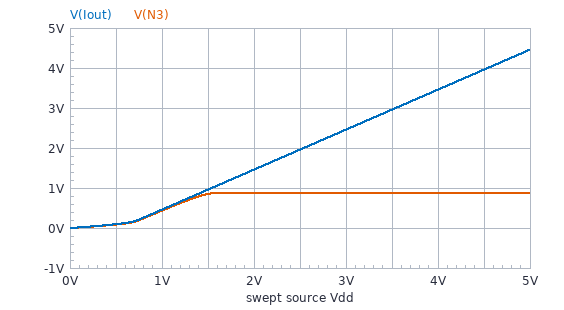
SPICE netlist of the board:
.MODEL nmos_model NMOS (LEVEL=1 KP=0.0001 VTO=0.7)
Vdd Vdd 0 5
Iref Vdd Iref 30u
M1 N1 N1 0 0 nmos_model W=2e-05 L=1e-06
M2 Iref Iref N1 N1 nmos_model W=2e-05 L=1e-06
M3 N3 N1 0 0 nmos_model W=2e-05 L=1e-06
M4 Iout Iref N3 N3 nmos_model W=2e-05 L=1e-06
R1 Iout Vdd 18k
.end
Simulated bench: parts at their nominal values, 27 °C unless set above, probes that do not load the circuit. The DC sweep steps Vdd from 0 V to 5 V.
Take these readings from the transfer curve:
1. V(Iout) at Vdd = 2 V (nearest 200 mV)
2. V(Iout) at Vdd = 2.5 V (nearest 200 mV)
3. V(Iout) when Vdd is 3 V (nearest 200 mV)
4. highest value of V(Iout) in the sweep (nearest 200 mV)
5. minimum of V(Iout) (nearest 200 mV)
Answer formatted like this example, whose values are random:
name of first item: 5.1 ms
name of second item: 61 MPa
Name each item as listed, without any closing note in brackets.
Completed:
V(Iout) at Vdd = 2 V: 1.4 V
V(Iout) at Vdd = 2.5 V: 2.0 V
V(Iout) when Vdd is 3 V: 2.4 V
highest value of V(Iout) in the sweep: 4.4 V
minimum of V(Iout): 0 V
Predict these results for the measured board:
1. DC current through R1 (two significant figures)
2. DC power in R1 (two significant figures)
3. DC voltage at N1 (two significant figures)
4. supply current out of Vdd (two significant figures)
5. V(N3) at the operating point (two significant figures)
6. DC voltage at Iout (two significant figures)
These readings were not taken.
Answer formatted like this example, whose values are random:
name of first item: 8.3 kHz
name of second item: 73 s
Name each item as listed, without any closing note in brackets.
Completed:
DC current through R1: 30 µA
DC power in R1: 16 µW
DC voltage at N1: 870 mV
supply current out of Vdd: 60 µA
V(N3) at the operating point: 870 mV
DC voltage at Iout: 4.5 V
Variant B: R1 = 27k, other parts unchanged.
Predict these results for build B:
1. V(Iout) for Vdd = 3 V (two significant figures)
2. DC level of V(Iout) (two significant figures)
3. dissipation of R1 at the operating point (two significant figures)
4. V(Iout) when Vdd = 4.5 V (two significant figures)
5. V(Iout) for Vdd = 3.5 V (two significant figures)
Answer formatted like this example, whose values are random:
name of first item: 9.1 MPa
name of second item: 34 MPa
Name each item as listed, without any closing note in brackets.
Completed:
V(Iout) for Vdd = 3 V: 2.2 V
DC level of V(Iout): 4.2 V
dissipation of R1 at the operating point: 24 µW
V(Iout) when Vdd = 4.5 V: 3.7 V
V(Iout) for Vdd = 3.5 V: 2.7 V
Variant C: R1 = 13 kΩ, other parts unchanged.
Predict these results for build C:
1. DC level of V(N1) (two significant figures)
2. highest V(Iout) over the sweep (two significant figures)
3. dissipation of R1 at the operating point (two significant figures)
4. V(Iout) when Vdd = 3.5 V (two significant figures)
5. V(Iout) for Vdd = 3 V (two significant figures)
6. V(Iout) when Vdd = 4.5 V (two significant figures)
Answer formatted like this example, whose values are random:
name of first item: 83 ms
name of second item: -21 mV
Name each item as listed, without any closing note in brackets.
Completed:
DC level of V(N1): 870 mV
highest V(Iout) over the sweep: 4.6 V
dissipation of R1 at the operating point: 12 µW
V(Iout) when Vdd = 3.5 V: 3.1 V
V(Iout) for Vdd = 3 V: 2.6 V
V(Iout) when Vdd = 4.5 V: 4.1 V
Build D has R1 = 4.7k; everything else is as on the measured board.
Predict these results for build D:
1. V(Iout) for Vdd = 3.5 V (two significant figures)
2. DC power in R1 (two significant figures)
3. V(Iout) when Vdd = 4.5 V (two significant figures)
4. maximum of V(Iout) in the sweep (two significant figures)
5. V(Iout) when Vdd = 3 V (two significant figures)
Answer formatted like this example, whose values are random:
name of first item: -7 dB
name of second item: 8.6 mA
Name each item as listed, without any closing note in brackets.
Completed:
V(Iout) for Vdd = 3.5 V: 3.4 V
DC power in R1: 4.2 µW
V(Iout) when Vdd = 4.5 V: 4.4 V
maximum of V(Iout) in the sweep: 4.9 V
V(Iout) when Vdd = 3 V: 2.9 V
